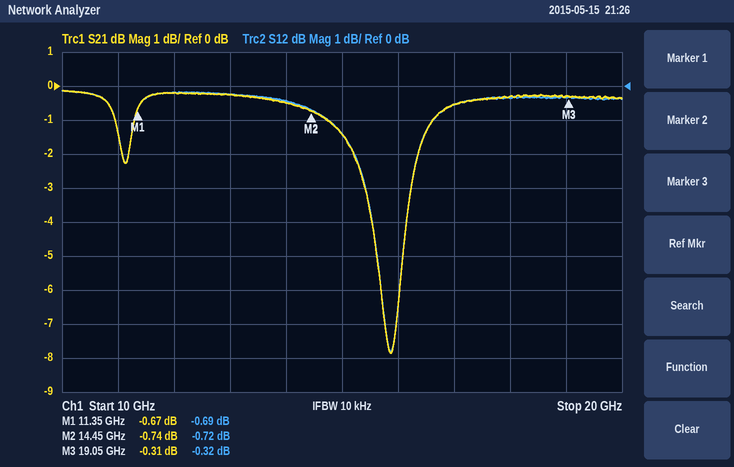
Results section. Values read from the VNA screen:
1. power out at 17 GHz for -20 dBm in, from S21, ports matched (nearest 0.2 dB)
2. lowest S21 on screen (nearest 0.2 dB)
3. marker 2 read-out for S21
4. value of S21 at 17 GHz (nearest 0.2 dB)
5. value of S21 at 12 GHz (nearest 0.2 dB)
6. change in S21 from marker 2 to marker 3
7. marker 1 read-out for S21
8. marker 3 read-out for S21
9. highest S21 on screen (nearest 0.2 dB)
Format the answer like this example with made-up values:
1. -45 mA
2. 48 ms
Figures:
1. -20.6 dBm
2. -7.8 dB
3. -0.74 dB
4. -0.6 dB
5. -0.2 dB
6. 0.43 dB
7. -0.67 dB
8. -0.31 dB
9. -0.2 dB
